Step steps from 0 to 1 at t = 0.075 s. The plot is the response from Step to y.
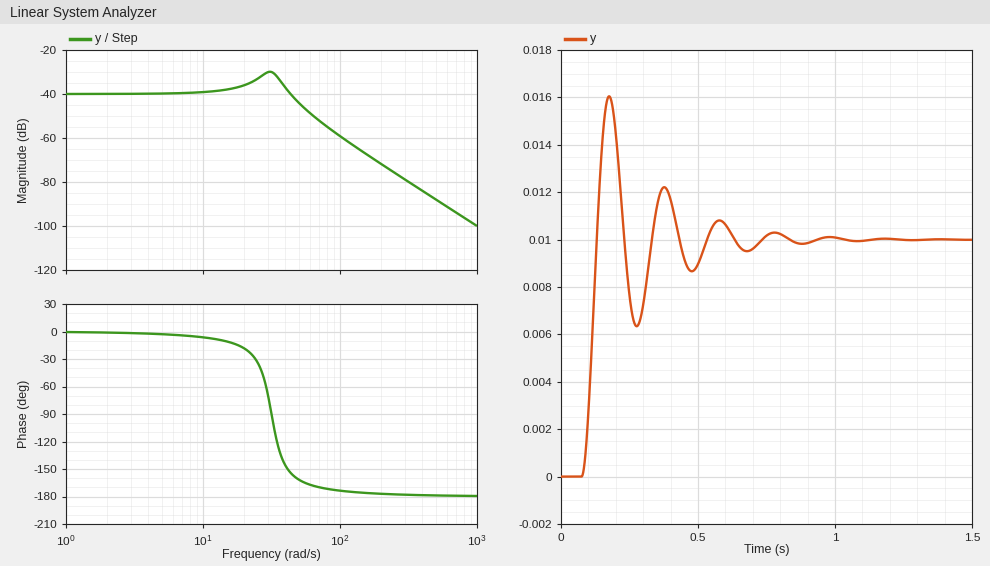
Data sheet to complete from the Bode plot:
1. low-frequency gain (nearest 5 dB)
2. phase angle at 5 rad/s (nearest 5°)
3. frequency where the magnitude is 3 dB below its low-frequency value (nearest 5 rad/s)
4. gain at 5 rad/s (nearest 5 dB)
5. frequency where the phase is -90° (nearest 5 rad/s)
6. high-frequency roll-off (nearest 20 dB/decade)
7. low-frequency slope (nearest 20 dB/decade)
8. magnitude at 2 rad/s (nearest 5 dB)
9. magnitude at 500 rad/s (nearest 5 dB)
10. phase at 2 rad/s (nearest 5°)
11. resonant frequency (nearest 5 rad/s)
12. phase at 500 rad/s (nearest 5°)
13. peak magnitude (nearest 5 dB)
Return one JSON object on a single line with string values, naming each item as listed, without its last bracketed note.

{"low-frequency gain": "-40 dB", "phase angle at 5 rad/s": "-5°", "frequency where the magnitude is 3 dB below its low-frequency value": "50 rad/s", "gain at 5 rad/s": "-40 dB", "frequency where the phase is -90°": "30 rad/s", "high-frequency roll-off": "-40 dB/decade", "low-frequency slope": "0 dB/decade", "magnitude at 2 rad/s": "-40 dB", "magnitude at 500 rad/s": "-90 dB", "phase at 2 rad/s": "0°", "resonant frequency": "30 rad/s", "phase at 500 rad/s": "-180°", "peak magnitude": "-30 dB"}
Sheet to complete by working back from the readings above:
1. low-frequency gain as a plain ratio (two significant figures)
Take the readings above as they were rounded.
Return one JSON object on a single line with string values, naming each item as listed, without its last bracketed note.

{"low-frequency gain as a plain ratio": "0.010"}
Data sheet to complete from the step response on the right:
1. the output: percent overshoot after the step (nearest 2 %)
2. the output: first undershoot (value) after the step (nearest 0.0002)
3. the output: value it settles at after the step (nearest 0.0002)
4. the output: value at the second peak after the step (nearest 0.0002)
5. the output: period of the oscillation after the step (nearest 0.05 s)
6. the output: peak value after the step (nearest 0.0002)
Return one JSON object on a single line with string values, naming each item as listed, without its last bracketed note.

{"the output: percent overshoot after the step": "60 %", "the output: first undershoot (value) after the step": "0.0064", "the output: value it settles at after the step": "0.0100", "the output: value at the second peak after the step": "0.0122", "the output: period of the oscillation after the step": "0.20 s", "the output: peak value after the step": "0.0160"}
